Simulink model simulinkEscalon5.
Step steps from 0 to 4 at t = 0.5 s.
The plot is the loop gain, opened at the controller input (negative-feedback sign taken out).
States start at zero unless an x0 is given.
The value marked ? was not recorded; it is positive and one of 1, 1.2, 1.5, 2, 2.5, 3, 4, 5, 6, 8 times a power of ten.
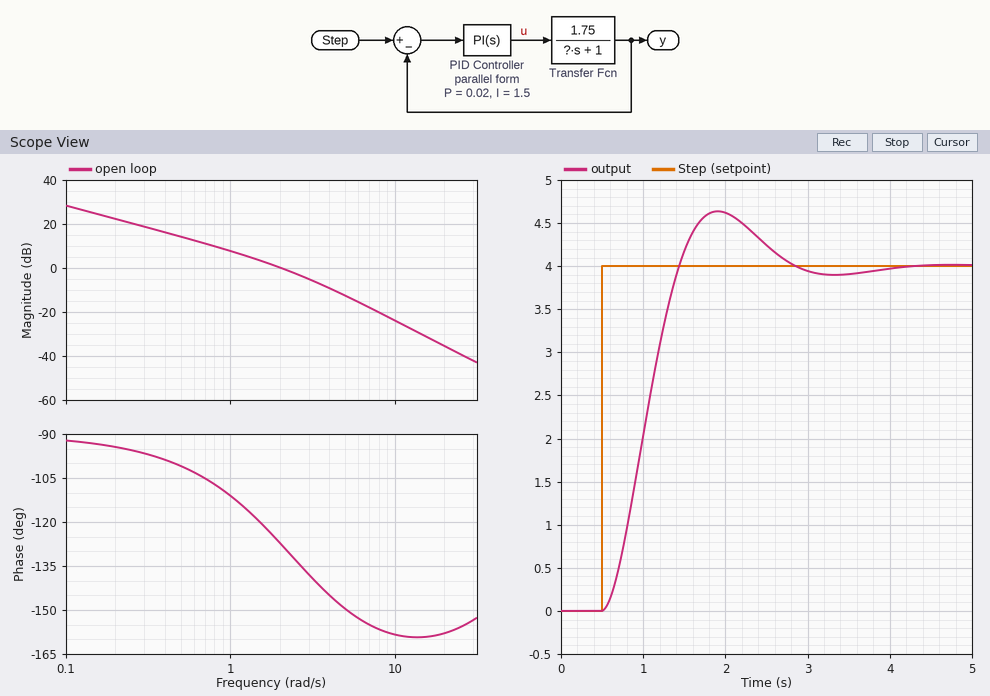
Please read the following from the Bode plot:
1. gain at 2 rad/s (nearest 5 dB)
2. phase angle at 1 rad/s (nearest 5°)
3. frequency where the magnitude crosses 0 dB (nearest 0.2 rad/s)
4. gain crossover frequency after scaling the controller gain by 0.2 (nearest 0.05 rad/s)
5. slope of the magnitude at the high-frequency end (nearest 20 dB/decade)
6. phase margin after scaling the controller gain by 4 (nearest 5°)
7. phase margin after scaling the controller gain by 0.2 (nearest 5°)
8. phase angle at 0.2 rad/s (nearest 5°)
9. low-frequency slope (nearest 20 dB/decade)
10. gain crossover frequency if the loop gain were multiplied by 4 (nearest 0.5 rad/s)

0 dB
-110°
2.0 rad/s
0.50 rad/s
-40 dB/decade
30°
80°
-95°
-20 dB/decade
5.0 rad/s
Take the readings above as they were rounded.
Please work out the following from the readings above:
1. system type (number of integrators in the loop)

1
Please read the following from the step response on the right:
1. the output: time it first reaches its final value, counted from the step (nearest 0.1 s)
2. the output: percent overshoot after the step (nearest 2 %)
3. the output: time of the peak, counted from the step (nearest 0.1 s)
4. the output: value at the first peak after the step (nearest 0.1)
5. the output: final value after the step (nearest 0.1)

0.9 s
16 %
1.4 s
4.6
4.0
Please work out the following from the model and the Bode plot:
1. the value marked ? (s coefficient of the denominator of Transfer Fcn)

0.4
